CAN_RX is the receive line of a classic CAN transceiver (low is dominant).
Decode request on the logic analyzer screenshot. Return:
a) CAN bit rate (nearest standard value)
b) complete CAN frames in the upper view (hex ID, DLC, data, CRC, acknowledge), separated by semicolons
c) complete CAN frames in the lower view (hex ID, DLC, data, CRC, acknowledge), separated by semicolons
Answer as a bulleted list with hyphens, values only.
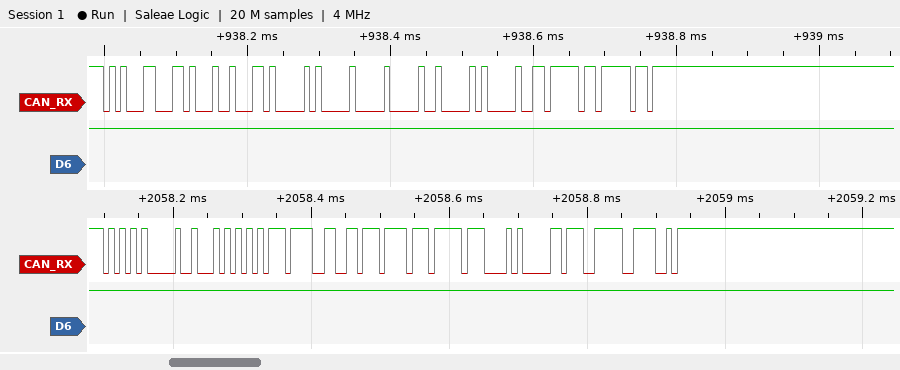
- 125 kbit/s
- ID 14611234, DLC 4, data 00 01 02 03, CRC 3FBF, ACK
- ID 550, DLC 8, data AA BB CC DD EE FF 0A 0B, CRC 4FBC, ACK
